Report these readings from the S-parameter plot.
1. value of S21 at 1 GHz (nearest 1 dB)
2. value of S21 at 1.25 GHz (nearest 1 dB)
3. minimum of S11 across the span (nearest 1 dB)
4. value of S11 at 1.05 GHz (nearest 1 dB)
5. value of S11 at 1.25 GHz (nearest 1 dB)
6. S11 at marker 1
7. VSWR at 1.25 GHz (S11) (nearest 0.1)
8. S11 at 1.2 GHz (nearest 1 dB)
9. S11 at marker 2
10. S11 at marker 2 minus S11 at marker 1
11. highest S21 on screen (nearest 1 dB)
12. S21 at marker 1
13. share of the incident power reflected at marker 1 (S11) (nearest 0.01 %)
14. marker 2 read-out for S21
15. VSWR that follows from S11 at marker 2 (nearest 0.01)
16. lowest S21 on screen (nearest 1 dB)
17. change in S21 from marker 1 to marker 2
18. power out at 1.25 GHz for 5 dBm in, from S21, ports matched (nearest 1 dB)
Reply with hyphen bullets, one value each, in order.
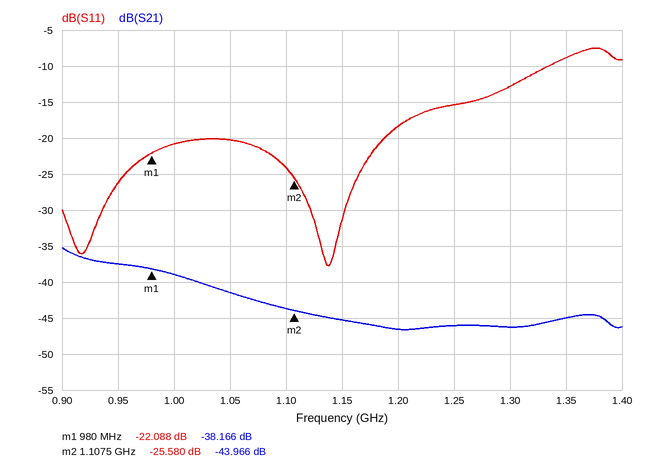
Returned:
- -39 dB
- -46 dB
- -38 dB
- -20 dB
- -15 dB
- -22.088 dB
- 1.4
- -18 dB
- -25.580 dB
- -3.492 dB
- -35 dB
- -38.166 dB
- 0.62 %
- -43.966 dB
- 1.11
- -47 dB
- -5.800 dB
- -41 dBm
